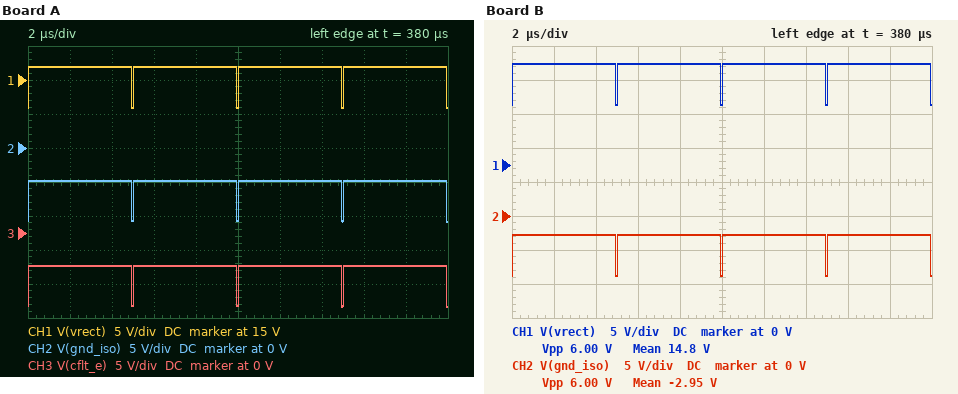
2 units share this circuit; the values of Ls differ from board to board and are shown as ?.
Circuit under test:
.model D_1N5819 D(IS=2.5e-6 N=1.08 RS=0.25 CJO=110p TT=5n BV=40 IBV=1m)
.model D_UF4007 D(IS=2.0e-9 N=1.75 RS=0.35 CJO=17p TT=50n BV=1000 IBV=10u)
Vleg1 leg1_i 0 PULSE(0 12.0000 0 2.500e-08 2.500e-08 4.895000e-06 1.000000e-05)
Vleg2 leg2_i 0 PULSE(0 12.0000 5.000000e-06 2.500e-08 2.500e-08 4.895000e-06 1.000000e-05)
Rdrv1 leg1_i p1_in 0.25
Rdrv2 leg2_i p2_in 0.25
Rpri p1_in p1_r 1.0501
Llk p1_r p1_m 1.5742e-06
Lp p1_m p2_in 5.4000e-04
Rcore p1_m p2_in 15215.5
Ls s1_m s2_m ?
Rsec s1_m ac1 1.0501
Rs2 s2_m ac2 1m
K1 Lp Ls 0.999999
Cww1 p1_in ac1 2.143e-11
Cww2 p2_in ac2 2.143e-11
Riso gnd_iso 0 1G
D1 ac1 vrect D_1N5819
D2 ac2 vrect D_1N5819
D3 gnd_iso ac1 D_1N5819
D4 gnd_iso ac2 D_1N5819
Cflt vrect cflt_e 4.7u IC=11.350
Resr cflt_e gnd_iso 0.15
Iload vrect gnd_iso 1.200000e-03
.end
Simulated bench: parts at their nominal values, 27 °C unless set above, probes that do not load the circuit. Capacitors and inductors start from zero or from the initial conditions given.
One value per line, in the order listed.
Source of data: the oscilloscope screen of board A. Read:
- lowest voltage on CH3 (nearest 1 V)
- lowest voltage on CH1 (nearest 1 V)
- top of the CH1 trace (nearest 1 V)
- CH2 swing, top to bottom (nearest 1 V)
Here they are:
-11 V
11 V
17 V
6 V
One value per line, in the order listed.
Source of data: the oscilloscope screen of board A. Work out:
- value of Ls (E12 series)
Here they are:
1.8 mH
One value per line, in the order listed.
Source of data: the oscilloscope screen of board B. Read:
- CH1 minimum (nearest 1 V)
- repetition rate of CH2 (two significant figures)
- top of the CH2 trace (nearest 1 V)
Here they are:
9 V
200 kHz
-3 V
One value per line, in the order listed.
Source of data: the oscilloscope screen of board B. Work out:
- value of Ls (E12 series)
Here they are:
1.2 mH
